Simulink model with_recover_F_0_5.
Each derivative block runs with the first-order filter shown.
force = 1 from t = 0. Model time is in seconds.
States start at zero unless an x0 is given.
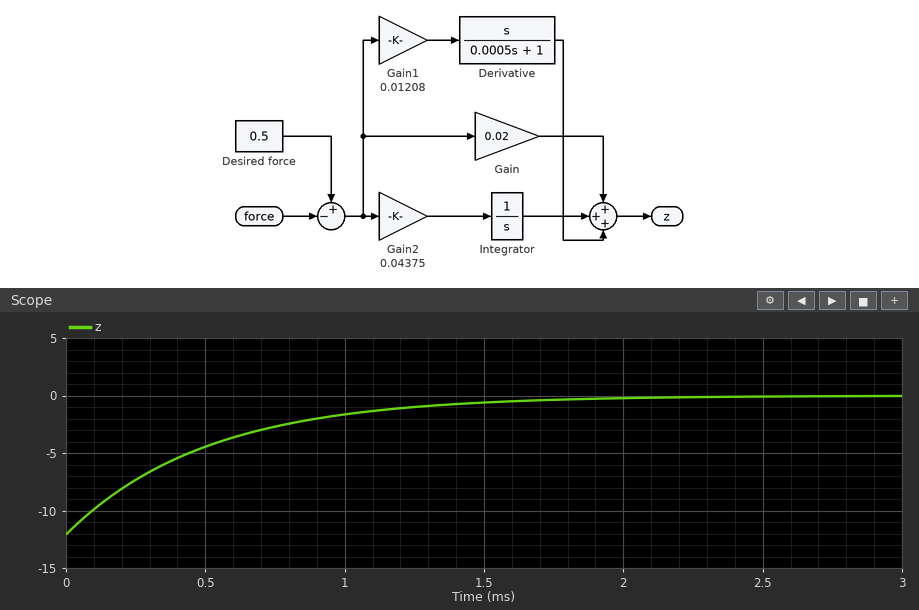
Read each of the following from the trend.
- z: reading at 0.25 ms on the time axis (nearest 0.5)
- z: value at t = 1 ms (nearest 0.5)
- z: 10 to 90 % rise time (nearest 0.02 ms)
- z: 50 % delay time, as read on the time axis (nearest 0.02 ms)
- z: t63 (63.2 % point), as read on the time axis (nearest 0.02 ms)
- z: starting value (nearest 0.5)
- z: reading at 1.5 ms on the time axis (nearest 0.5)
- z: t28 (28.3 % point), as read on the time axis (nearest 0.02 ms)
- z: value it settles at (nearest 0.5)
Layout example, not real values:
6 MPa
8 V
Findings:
-7.5
-1.5
1.10 ms
0.34 ms
0.50 ms
-12.0
-0.5
0.16 ms
0.0
